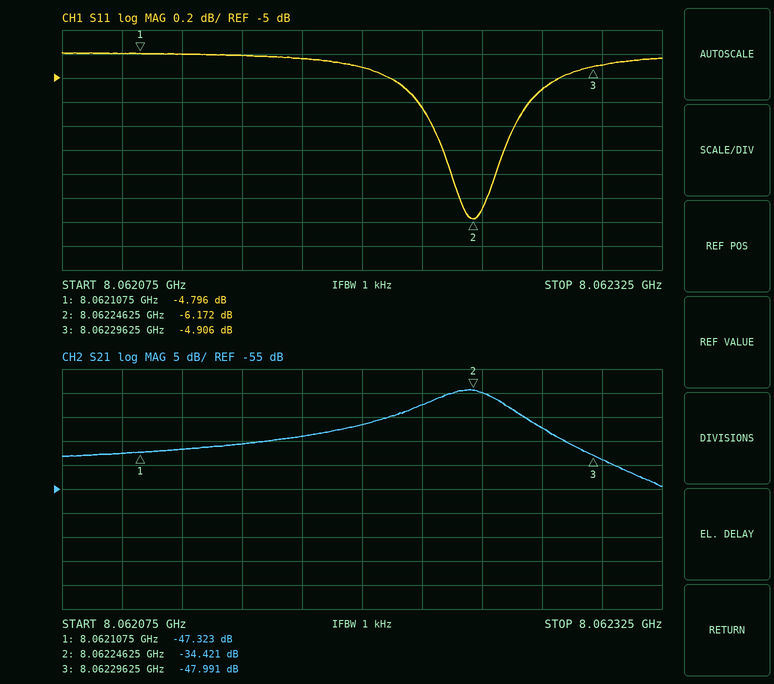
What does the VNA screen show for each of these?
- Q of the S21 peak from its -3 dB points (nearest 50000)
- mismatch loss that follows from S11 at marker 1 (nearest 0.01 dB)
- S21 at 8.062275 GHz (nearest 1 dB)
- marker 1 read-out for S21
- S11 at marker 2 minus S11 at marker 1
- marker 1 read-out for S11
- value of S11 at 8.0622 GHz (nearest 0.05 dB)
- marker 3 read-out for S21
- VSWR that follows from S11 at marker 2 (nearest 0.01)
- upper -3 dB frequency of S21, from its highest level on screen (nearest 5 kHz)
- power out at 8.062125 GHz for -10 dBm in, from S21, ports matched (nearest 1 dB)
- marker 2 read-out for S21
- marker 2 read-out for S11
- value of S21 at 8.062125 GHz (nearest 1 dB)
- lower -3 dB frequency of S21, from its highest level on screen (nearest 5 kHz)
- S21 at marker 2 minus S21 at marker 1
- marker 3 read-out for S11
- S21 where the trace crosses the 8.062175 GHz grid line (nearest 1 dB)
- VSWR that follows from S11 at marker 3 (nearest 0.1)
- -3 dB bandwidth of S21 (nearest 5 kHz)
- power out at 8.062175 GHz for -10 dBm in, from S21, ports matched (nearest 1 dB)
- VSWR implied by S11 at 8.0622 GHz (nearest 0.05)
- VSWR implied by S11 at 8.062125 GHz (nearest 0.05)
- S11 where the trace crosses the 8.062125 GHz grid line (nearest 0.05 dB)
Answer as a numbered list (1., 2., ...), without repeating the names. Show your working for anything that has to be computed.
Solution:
1. 8.06224 GHz / 35 kHz ≈ 230350, so 250000 to the nearest 50000
2. −10 log10(1 − 10^(-4.796/10)) ≈ 1.75 dB
3. -42 dB
4. -47.323 dB
5. -6.172 − (-4.796) = -1.376 dB
6. -4.796 dB
7. -4.90 dB
8. -47.991 dB
9. (1 + 0.4914)/(1 − 0.4914) ≈ 2.93
10. 8.062260 GHz
11. -10 dBm + (-47 dB) = -57 dBm
12. -34.421 dB
13. -6.172 dB
14. -47 dB
15. 8.062225 GHz
16. -34.421 − (-47.323) = 12.902 dB
17. -4.906 dB
18. -44 dB
19. (1 + 0.5685)/(1 − 0.5685) ≈ 3.6
20. 8.062260 GHz − 8.062225 GHz = 35 kHz
21. -10 dBm + (-44 dB) = -54 dBm
22. |Γ| = 10^(-4.9/20) = 0.5689; VSWR = (1 + 0.5689)/(1 − 0.5689) ≈ 3.64, so 3.65 to the nearest 0.05
23. |Γ| = 10^(-4.8/20) = 0.5754; VSWR = (1 + 0.5754)/(1 − 0.5754) ≈ 3.71, so 3.70 to the nearest 0.05
24. -4.80 dB
